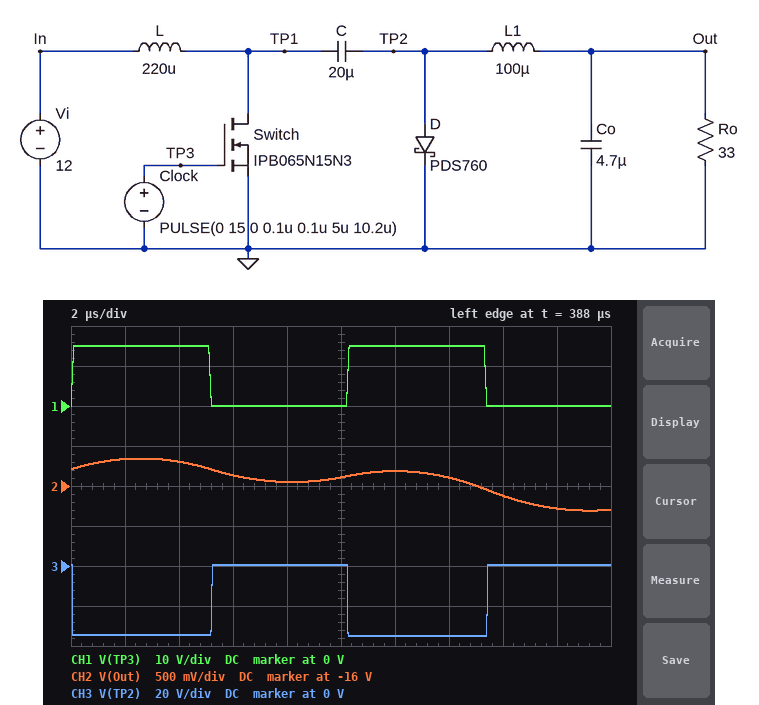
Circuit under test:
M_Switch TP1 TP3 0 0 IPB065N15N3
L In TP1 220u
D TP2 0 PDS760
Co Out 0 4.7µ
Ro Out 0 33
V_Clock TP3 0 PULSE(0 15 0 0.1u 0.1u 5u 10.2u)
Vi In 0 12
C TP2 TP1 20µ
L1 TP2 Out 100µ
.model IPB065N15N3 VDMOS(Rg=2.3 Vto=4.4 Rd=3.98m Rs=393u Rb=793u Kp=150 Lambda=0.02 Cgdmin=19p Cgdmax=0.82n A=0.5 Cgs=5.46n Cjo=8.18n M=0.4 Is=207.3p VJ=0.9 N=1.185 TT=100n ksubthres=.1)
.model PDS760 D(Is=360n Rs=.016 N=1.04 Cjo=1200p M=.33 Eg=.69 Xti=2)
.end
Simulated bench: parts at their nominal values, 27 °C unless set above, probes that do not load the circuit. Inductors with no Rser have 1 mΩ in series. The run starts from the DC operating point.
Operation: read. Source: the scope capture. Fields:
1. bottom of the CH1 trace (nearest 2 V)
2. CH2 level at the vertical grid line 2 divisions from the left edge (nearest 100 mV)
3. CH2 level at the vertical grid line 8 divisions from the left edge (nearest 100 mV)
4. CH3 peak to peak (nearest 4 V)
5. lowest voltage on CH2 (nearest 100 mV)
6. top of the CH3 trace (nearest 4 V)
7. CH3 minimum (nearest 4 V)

0 V
-15.7 V
-16.1 V
36 V
-16.3 V
0 V
-36 V
